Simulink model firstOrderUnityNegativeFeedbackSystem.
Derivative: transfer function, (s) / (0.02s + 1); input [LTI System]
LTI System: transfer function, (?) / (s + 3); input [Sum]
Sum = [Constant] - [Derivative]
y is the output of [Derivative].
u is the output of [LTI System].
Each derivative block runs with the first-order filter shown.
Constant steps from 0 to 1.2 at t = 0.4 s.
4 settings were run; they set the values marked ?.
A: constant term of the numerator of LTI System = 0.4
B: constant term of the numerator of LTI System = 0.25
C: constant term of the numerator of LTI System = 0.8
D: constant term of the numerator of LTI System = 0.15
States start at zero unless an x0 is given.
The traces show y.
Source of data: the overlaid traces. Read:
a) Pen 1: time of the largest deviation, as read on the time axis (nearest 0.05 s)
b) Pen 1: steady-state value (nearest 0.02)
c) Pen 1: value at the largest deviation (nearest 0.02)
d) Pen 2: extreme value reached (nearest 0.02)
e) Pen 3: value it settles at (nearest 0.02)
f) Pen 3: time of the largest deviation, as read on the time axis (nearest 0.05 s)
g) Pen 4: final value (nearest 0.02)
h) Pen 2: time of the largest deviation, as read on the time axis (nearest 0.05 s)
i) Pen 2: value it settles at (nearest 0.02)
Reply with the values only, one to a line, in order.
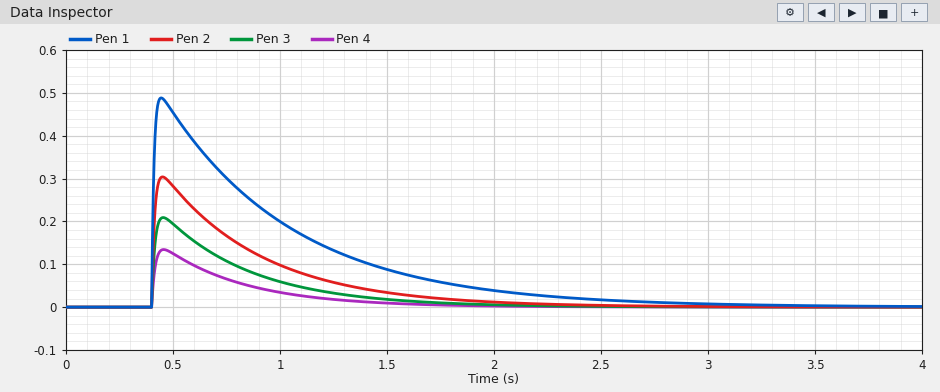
0.45 s
0.00
0.48
0.30
0.00
0.45 s
0.00
0.45 s
0.00
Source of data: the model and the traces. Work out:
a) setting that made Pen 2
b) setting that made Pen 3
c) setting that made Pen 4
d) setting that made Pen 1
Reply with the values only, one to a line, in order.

A
B
D
C
